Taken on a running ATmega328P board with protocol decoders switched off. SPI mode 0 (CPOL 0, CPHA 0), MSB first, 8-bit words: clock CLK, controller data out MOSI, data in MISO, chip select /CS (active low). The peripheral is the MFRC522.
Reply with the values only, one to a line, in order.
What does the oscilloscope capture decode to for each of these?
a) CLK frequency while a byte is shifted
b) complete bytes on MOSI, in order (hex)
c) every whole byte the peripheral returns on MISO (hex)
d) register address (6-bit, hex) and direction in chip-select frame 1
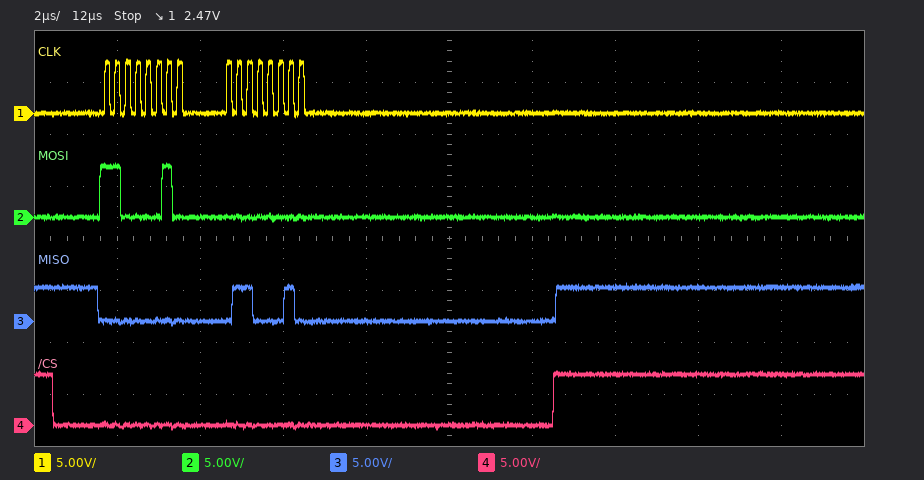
4 MHz
C2 00
00 62
0x21 read
